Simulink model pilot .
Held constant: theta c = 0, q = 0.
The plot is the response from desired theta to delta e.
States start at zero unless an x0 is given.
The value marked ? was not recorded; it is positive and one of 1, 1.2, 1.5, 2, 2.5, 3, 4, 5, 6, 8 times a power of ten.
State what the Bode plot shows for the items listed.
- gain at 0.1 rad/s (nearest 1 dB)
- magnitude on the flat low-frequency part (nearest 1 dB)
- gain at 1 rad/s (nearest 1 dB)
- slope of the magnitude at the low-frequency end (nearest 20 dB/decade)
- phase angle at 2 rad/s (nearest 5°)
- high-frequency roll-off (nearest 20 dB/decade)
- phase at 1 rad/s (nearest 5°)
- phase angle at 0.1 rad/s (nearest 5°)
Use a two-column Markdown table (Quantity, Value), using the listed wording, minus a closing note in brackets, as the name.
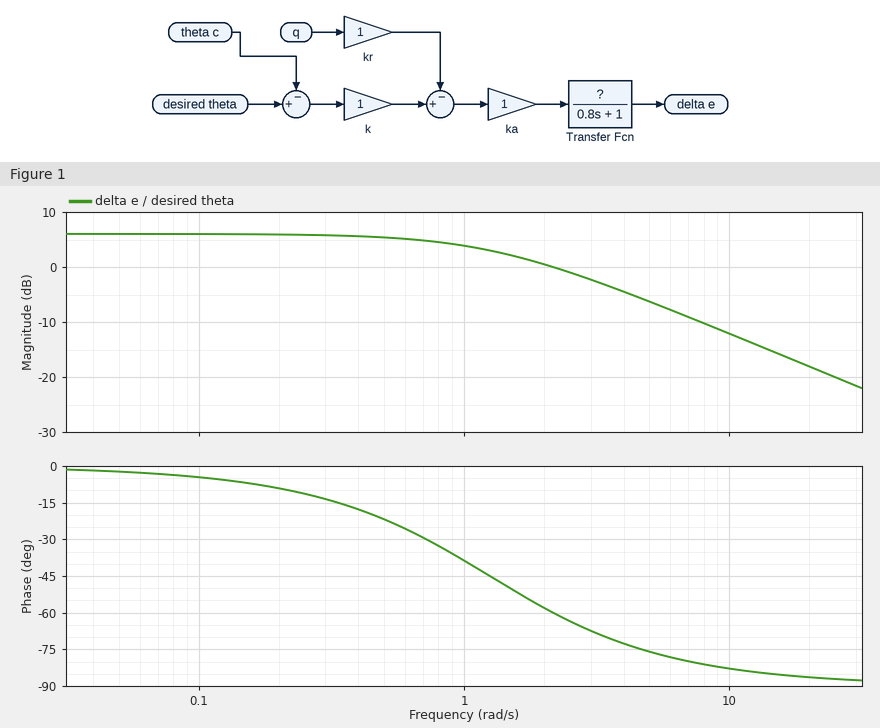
| Quantity | Value |
|---|---|
| gain at 0.1 rad/s | 6 dB |
| magnitude on the flat low-frequency part | 6 dB |
| gain at 1 rad/s | 4 dB |
| slope of the magnitude at the low-frequency end | 0 dB/decade |
| phase angle at 2 rad/s | -60° |
| high-frequency roll-off | -20 dB/decade |
| phase at 1 rad/s | -40° |
| phase angle at 0.1 rad/s | -5° |
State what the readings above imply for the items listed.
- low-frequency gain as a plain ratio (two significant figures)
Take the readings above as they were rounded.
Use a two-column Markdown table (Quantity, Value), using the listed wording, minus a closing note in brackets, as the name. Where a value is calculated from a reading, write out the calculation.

| Quantity | Value |
|---|---|
| low-frequency gain as a plain ratio | 10^(6 / 20) = 2.0 |
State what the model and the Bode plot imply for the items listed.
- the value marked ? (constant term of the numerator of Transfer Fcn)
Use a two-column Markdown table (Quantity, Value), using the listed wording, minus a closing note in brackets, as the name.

| Quantity | Value |
|---|---|
| the value marked ? | 2 |
